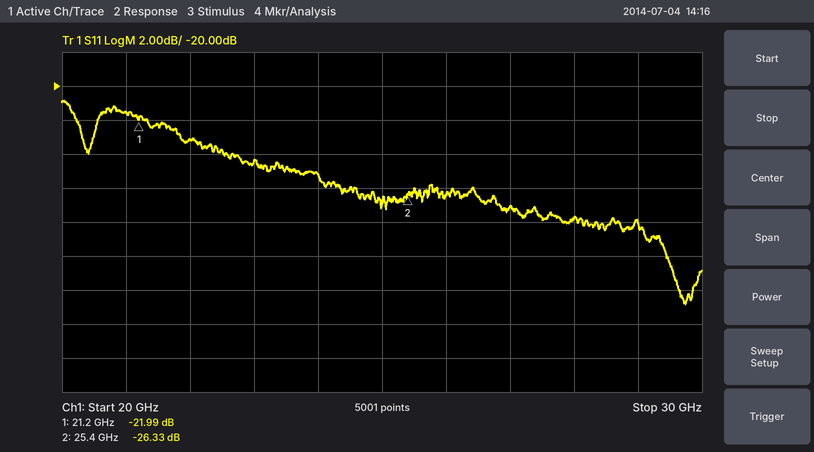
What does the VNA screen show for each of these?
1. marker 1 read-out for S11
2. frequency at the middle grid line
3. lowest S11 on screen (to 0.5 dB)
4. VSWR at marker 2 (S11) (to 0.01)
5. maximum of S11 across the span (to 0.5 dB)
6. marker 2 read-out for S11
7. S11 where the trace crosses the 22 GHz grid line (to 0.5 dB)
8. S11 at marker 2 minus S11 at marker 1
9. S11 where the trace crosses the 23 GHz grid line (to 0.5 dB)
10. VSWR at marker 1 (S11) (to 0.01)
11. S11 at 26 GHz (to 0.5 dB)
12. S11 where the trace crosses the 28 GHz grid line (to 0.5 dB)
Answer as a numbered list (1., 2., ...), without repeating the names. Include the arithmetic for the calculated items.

1. -21.99 dB
2. 25 GHz
3. -33.0 dB
4. (1 + 0.0483)/(1 − 0.0483) ≈ 1.10
5. -21.0 dB
6. -26.33 dB
7. -23.0 dB
8. -26.33 − (-21.99) = -4.34 dB
9. -24.5 dB
10. (1 + 0.0795)/(1 − 0.0795) ≈ 1.17
11. -26.5 dB
12. -28.0 dB
